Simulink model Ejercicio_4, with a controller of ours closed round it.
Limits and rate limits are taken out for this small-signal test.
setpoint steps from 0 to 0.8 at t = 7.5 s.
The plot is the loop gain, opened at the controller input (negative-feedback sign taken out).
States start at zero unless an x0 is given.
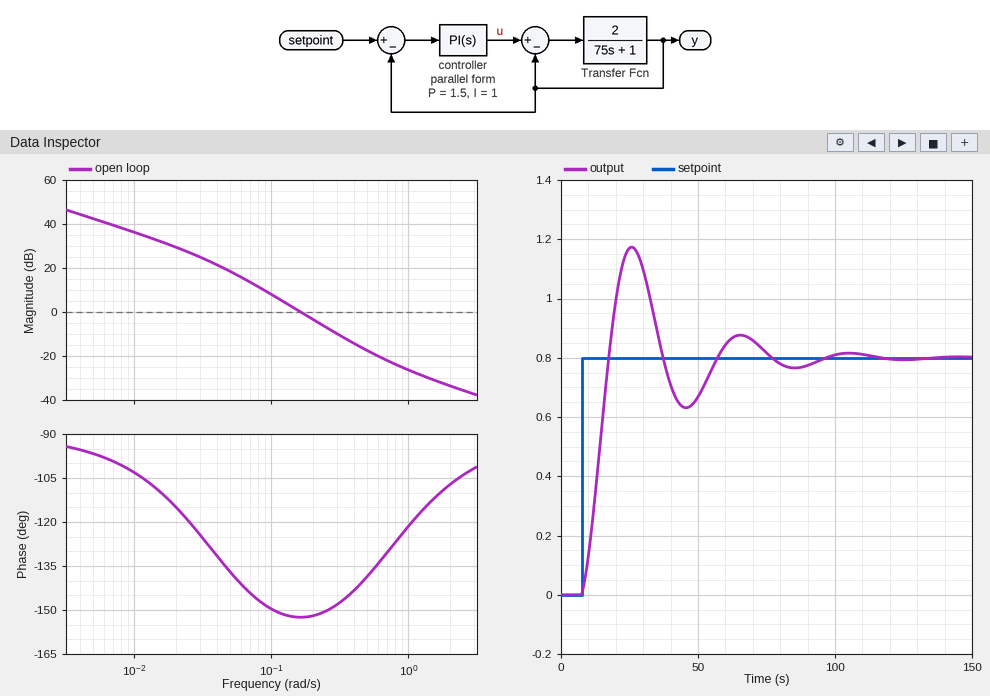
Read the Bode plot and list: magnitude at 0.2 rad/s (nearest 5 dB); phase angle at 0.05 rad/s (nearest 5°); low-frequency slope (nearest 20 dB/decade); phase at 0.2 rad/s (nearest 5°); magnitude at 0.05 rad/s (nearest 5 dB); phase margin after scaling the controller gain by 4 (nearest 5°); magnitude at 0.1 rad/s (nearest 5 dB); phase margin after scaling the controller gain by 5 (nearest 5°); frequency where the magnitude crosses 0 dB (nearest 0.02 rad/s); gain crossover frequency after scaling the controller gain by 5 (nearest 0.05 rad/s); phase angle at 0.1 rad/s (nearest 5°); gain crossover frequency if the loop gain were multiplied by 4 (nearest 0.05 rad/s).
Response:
-5 dB
-135°
-20 dB/decade
-150°
20 dB
35°
10 dB
35°
0.16 rad/s
0.40 rad/s
-150°
0.35 rad/s
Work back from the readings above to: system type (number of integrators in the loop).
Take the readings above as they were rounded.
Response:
1
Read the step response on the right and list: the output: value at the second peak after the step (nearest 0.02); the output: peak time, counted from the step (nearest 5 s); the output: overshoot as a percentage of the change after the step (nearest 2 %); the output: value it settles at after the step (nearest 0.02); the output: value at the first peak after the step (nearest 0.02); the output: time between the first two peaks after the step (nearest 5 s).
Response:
0.88
20 s
46 %
0.80
1.18
40 s
